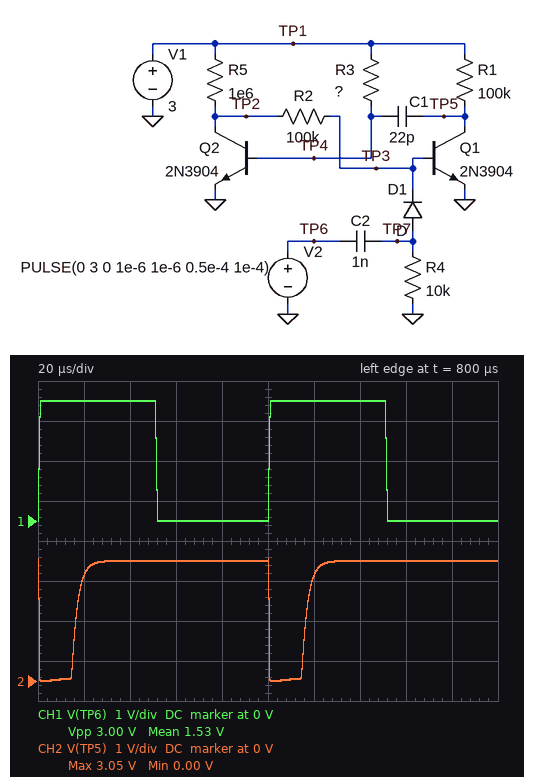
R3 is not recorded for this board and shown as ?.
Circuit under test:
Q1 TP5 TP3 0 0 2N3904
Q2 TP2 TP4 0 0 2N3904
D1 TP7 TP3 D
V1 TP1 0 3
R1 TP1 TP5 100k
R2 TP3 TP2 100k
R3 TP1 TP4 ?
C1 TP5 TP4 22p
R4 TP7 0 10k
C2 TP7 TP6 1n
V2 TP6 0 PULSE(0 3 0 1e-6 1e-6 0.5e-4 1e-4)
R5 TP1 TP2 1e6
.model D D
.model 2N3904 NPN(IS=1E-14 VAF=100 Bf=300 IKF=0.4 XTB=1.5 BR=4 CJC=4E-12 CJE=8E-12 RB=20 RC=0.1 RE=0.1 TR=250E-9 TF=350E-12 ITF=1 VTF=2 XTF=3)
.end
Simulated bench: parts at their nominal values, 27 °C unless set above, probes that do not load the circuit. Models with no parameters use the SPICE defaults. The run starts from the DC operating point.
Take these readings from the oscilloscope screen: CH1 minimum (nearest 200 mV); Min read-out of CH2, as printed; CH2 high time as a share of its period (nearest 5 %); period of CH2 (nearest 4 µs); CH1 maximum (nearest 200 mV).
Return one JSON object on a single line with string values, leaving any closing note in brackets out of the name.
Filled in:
{"CH1 minimum": "0 V", "Min read-out of CH2, as printed": "0.00 V", "CH2 high time as a share of its period": "85 %", "period of CH2": "100 µs", "CH1 maximum": "3.0 V"}
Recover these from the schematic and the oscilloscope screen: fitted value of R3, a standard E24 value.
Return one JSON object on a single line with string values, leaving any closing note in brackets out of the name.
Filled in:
{"fitted value of R3, a standard E24 value": "750 kΩ"}
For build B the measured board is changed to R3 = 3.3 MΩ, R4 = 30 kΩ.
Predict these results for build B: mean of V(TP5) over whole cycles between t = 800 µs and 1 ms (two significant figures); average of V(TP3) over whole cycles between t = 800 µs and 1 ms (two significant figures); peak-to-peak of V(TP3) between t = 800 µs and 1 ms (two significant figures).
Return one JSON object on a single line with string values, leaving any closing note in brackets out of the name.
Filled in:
{"mean of V(TP5) over whole cycles between t = 800 µs and 1 ms": "1.1 V", "average of V(TP3) over whole cycles between t = 800 µs and 1 ms": "380 mV", "peak-to-peak of V(TP3) between t = 800 µs and 1 ms": "740 mV"}
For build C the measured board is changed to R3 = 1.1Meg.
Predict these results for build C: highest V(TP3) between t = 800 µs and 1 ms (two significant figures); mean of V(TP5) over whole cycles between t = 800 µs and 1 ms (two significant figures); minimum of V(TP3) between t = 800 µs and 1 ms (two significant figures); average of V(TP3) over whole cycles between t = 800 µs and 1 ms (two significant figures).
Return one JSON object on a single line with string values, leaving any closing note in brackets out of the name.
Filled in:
{"highest V(TP3) between t = 800 µs and 1 ms": "760 mV", "mean of V(TP5) over whole cycles between t = 800 µs and 1 ms": "2.3 V", "minimum of V(TP3) between t = 800 µs and 1 ms": "12 mV", "average of V(TP3) over whole cycles between t = 800 µs and 1 ms": "150 mV"}
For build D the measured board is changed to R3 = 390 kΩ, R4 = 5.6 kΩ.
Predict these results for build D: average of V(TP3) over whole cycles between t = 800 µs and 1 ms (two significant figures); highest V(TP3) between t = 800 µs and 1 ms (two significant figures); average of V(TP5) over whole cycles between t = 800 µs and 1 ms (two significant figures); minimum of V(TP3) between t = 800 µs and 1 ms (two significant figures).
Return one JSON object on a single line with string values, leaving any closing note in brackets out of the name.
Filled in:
{"average of V(TP3) over whole cycles between t = 800 µs and 1 ms": "72 mV", "highest V(TP3) between t = 800 µs and 1 ms": "760 mV", "average of V(TP5) over whole cycles between t = 800 µs and 1 ms": "2.7 V", "minimum of V(TP3) between t = 800 µs and 1 ms": "8.2 mV"}
